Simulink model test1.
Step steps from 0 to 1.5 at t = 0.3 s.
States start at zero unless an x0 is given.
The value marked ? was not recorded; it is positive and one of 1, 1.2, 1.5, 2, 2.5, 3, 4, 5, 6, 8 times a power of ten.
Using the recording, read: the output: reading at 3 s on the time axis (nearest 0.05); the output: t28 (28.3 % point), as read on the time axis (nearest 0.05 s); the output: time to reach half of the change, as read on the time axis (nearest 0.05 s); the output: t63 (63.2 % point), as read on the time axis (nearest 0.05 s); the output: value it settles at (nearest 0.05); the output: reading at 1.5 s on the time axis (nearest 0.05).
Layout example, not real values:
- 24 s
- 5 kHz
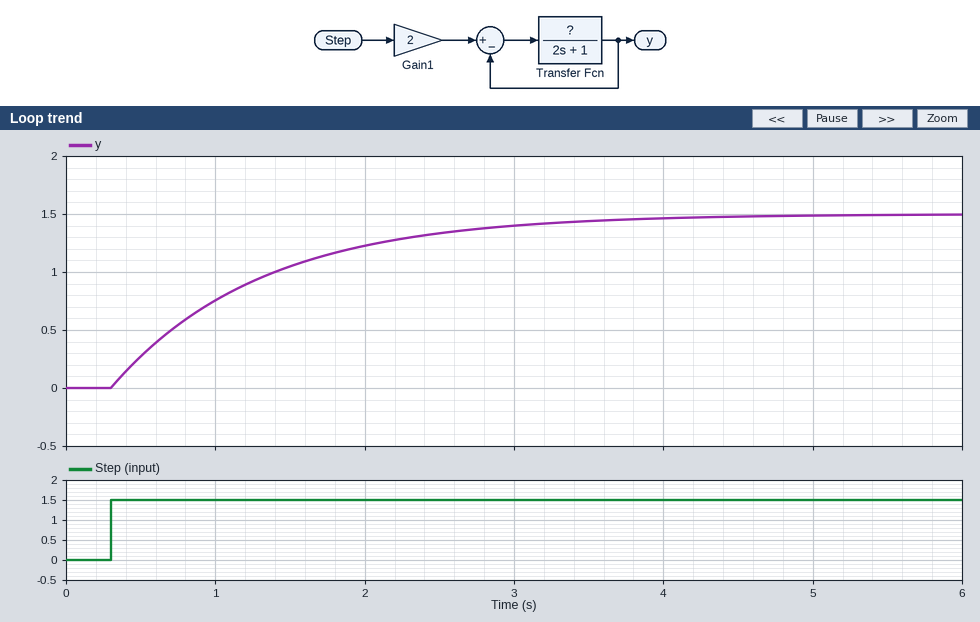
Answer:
- 1.40
- 0.65 s
- 1.00 s
- 1.30 s
- 1.50
- 1.05
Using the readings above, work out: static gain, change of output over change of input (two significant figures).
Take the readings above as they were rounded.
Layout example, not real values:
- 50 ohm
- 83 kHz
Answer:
- 1.0
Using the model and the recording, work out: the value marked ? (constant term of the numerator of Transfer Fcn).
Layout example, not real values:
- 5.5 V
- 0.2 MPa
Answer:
- 1
